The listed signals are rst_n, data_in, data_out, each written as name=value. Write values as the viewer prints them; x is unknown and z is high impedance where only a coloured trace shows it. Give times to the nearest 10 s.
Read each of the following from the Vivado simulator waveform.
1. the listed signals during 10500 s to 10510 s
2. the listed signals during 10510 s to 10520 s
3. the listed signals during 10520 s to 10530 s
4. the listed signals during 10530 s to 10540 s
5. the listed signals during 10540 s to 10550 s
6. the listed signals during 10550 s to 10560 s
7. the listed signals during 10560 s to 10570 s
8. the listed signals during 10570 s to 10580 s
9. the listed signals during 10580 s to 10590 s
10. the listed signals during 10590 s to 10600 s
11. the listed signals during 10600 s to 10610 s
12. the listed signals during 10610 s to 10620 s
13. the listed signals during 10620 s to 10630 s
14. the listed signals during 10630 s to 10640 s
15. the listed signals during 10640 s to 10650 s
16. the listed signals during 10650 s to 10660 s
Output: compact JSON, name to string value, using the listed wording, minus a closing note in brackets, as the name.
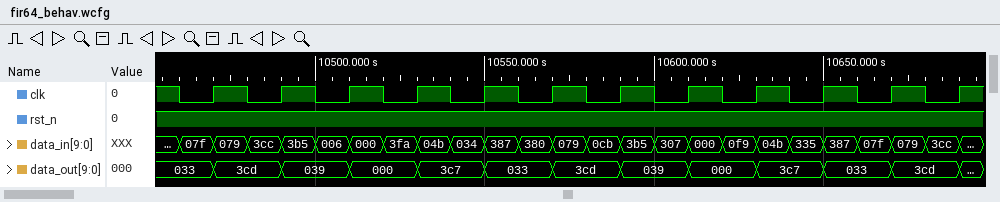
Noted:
{"the listed signals during 10500 s to 10510 s": "rst_n=1, data_in=006, data_out=039", "the listed signals during 10510 s to 10520 s": "rst_n=1, data_in=000, data_out=000", "the listed signals during 10520 s to 10530 s": "rst_n=1, data_in=3fa, data_out=000", "the listed signals during 10530 s to 10540 s": "rst_n=1, data_in=04b, data_out=3c7", "the listed signals during 10540 s to 10550 s": "rst_n=1, data_in=034, data_out=3c7", "the listed signals during 10550 s to 10560 s": "rst_n=1, data_in=387, data_out=033", "the listed signals during 10560 s to 10570 s": "rst_n=1, data_in=380, data_out=033", "the listed signals during 10570 s to 10580 s": "rst_n=1, data_in=079, data_out=3cd", "the listed signals during 10580 s to 10590 s": "rst_n=1, data_in=0cb, data_out=3cd", "the listed signals during 10590 s to 10600 s": "rst_n=1, data_in=3b5, data_out=039", "the listed signals during 10600 s to 10610 s": "rst_n=1, data_in=307, data_out=039", "the listed signals during 10610 s to 10620 s": "rst_n=1, data_in=000, data_out=000", "the listed signals during 10620 s to 10630 s": "rst_n=1, data_in=0f9, data_out=000", "the listed signals during 10630 s to 10640 s": "rst_n=1, data_in=04b, data_out=3c7", "the listed signals during 10640 s to 10650 s": "rst_n=1, data_in=335, data_out=3c7", "the listed signals during 10650 s to 10660 s": "rst_n=1, data_in=387, data_out=033"}
